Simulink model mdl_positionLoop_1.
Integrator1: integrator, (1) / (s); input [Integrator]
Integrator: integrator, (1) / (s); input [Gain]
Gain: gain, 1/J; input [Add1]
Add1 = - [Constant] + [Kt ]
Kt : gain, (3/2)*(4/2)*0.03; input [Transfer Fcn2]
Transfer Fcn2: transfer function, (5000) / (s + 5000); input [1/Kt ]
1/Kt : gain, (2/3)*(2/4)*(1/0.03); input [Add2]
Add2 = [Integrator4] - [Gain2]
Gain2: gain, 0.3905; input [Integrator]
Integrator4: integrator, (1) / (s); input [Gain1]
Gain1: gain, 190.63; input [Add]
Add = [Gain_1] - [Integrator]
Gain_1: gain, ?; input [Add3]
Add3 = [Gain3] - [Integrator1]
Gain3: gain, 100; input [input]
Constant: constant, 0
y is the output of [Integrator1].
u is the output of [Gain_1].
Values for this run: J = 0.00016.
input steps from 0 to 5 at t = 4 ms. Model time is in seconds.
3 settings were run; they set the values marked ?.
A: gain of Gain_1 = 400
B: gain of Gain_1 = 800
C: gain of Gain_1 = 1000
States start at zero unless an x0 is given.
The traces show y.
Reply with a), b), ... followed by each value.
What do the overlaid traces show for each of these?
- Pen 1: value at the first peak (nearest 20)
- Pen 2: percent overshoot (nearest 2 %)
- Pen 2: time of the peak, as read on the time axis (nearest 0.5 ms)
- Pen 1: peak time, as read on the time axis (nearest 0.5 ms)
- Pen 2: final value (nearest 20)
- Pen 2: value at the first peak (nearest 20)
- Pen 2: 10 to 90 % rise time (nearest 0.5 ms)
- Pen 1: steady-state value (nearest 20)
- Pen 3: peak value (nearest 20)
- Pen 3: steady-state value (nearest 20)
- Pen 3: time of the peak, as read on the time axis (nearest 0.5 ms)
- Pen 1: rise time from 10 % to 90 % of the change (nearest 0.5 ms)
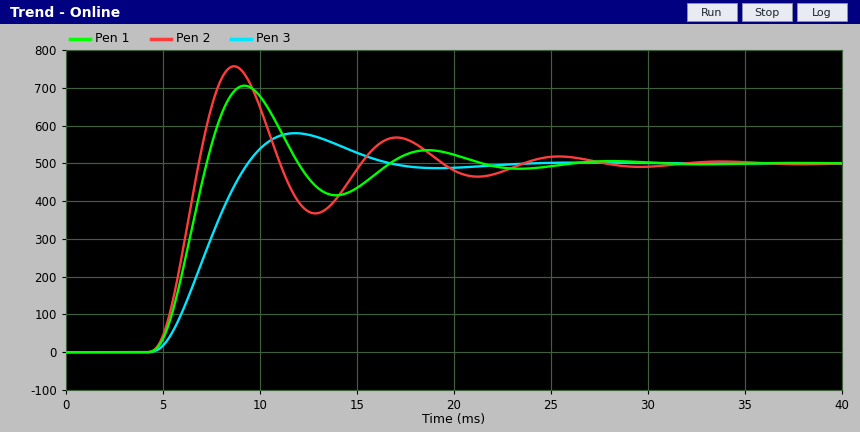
a) 700
b) 52 %
c) 8.5 ms
d) 9.0 ms
e) 500
f) 760
g) 1.5 ms
h) 500
i) 580
j) 500
k) 12.0 ms
l) 2.0 ms
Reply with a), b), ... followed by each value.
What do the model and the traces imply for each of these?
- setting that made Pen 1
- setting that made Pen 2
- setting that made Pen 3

a) B
b) C
c) A
